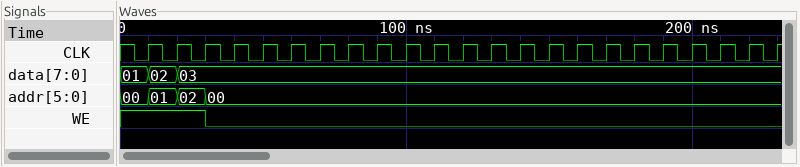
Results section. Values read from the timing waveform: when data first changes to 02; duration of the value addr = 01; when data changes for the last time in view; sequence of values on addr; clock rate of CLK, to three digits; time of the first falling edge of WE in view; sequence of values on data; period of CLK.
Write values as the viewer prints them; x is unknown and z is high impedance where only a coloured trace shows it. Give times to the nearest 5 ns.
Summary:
10 ns
10 ns
20 ns
00, 01, 02, 00
100 MHz
30 ns
01, 02, 03
10 ns
